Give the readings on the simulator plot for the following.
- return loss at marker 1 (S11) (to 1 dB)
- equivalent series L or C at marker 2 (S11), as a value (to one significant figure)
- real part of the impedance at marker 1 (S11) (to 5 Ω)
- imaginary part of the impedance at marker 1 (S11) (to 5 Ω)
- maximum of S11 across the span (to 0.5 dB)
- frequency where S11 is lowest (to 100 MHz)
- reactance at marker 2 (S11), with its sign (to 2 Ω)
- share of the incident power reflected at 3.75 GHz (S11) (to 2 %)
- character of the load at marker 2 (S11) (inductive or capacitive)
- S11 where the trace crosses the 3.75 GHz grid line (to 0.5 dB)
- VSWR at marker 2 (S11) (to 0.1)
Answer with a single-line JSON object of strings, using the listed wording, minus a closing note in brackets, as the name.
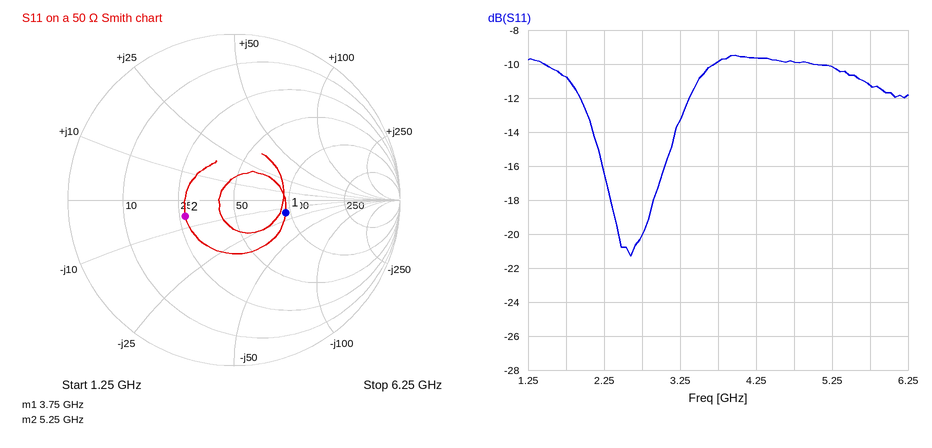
{"return loss at marker 1 (S11)": "10 dB", "equivalent series L or C at marker 2 (S11), as a value": "5 pF", "real part of the impedance at marker 1 (S11)": "95 Ω", "imaginary part of the impedance at marker 1 (S11)": "-15 Ω", "maximum of S11 across the span": "-9.5 dB", "frequency where S11 is lowest": "2.6 GHz", "reactance at marker 2 (S11), with its sign": "-6 Ω", "share of the incident power reflected at 3.75 GHz (S11)": "10 %", "character of the load at marker 2 (S11)": "capacitive", "S11 where the trace crosses the 3.75 GHz grid line": "-10.0 dB", "VSWR at marker 2 (S11)": "1.9"}
